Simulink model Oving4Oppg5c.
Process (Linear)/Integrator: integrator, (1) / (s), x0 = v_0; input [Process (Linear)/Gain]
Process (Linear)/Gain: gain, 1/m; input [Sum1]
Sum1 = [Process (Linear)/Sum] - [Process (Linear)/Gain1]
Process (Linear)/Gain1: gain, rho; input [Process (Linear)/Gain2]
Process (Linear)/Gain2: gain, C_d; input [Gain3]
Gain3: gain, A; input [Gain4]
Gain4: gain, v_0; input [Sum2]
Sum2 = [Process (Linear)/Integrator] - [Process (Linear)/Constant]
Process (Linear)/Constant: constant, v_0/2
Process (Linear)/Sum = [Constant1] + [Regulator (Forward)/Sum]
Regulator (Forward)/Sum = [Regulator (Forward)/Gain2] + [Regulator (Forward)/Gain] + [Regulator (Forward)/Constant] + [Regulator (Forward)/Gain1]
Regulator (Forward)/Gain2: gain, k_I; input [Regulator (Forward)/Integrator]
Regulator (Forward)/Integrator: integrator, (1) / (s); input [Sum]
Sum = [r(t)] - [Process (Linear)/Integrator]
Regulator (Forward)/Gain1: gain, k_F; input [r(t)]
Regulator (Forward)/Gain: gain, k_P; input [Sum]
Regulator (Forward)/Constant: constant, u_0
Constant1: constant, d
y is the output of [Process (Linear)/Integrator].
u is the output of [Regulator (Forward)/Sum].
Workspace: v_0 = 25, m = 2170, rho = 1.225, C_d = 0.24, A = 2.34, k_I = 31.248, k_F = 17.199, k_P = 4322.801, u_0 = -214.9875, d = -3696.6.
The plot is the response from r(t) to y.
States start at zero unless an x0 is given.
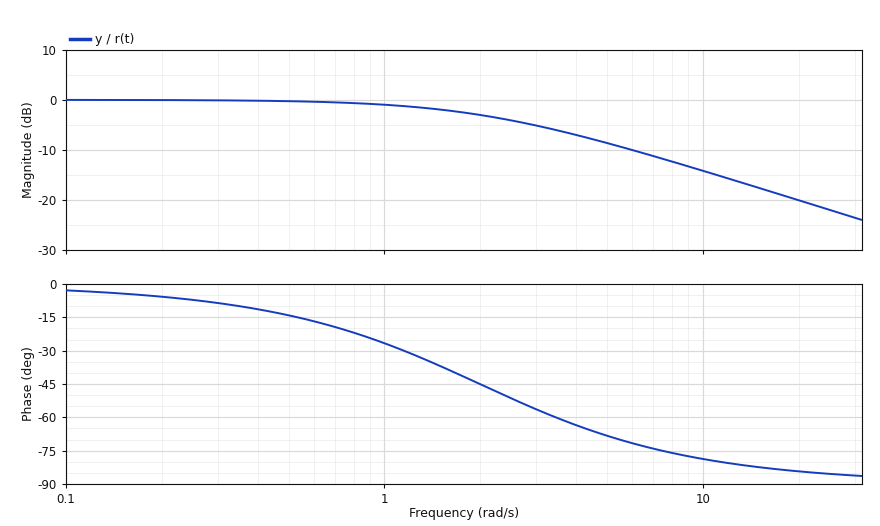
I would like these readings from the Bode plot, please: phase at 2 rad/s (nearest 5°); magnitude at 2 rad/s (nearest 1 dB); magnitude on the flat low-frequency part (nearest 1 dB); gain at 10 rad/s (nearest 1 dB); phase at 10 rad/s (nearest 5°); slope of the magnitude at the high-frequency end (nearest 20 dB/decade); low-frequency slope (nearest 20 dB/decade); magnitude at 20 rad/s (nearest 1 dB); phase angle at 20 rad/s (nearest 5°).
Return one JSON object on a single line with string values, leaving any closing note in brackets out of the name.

{"phase at 2 rad/s": "-45°", "magnitude at 2 rad/s": "-3 dB", "magnitude on the flat low-frequency part": "0 dB", "gain at 10 rad/s": "-14 dB", "phase at 10 rad/s": "-80°", "slope of the magnitude at the high-frequency end": "-20 dB/decade", "low-frequency slope": "0 dB/decade", "magnitude at 20 rad/s": "-20 dB", "phase angle at 20 rad/s": "-85°"}
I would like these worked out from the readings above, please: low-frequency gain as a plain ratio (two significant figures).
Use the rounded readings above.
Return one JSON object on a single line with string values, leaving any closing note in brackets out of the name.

{"low-frequency gain as a plain ratio": "1.0"}
